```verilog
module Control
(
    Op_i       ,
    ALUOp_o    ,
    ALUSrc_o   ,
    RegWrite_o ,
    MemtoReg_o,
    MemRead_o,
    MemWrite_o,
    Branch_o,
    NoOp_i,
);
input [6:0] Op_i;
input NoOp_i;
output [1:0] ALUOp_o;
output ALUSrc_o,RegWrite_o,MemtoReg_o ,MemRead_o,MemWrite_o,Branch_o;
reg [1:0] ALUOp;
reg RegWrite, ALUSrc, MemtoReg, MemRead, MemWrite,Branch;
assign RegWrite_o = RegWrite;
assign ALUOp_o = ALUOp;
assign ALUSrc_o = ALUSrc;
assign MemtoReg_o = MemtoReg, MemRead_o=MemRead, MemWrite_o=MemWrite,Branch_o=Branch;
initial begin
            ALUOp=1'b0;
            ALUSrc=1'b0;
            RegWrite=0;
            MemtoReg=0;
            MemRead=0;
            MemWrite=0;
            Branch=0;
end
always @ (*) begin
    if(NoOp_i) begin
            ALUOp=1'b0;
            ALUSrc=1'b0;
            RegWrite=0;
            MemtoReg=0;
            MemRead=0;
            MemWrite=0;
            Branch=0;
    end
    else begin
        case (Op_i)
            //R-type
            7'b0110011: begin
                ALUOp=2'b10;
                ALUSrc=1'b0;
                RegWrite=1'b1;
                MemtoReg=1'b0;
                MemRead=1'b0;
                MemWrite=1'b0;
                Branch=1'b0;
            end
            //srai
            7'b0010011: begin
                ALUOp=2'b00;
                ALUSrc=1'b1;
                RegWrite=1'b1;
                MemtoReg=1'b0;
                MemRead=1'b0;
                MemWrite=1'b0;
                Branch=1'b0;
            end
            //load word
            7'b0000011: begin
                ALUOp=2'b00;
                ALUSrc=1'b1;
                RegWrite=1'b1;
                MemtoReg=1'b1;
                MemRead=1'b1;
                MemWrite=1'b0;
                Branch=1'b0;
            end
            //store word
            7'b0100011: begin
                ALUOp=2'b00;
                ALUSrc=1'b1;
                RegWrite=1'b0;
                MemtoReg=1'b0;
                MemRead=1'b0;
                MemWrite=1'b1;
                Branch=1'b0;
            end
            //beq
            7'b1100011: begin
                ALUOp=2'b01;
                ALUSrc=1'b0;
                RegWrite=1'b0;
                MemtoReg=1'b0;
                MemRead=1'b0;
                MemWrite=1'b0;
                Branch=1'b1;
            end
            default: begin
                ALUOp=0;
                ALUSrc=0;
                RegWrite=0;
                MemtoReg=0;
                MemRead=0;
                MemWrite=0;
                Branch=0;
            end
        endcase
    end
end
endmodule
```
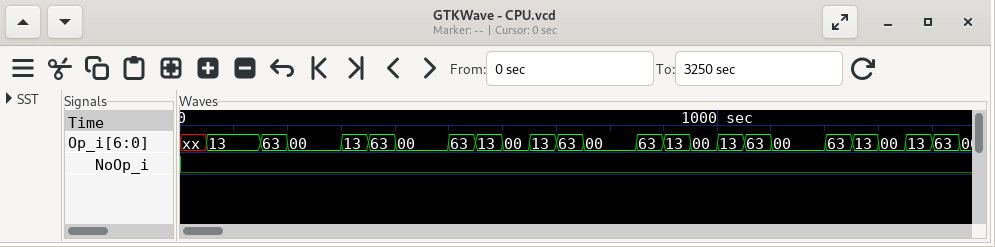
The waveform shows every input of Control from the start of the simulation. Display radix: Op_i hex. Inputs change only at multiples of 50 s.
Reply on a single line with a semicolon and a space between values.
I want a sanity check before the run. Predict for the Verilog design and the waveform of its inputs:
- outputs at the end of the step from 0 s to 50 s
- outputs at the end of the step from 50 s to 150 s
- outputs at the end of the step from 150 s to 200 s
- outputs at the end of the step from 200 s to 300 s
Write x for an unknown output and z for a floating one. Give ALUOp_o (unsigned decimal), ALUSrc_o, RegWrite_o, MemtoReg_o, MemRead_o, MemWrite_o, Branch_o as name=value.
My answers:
ALUOp_o=0, ALUSrc_o=0, RegWrite_o=0, MemtoReg_o=0, MemRead_o=0, MemWrite_o=0, Branch_o=0; ALUOp_o=0, ALUSrc_o=1, RegWrite_o=1, MemtoReg_o=0, MemRead_o=0, MemWrite_o=0, Branch_o=0; ALUOp_o=1, ALUSrc_o=0, RegWrite_o=0, MemtoReg_o=0, MemRead_o=0, MemWrite_o=0, Branch_o=1; ALUOp_o=0, ALUSrc_o=0, RegWrite_o=0, MemtoReg_o=0, MemRead_o=0, MemWrite_o=0, Branch_o=0
